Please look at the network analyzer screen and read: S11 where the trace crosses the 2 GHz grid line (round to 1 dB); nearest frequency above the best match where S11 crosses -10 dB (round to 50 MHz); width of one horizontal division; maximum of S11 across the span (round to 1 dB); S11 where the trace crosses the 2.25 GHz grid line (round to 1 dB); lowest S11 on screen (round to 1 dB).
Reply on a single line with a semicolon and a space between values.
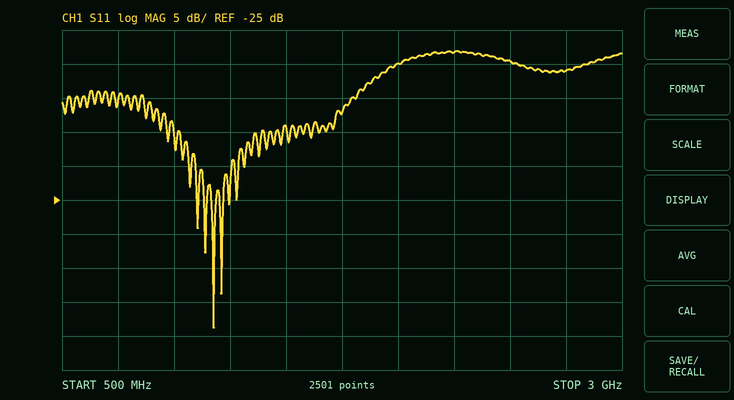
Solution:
-5 dB; 1.80 GHz; 250 MHz; -3 dB; -3 dB; -44 dB
